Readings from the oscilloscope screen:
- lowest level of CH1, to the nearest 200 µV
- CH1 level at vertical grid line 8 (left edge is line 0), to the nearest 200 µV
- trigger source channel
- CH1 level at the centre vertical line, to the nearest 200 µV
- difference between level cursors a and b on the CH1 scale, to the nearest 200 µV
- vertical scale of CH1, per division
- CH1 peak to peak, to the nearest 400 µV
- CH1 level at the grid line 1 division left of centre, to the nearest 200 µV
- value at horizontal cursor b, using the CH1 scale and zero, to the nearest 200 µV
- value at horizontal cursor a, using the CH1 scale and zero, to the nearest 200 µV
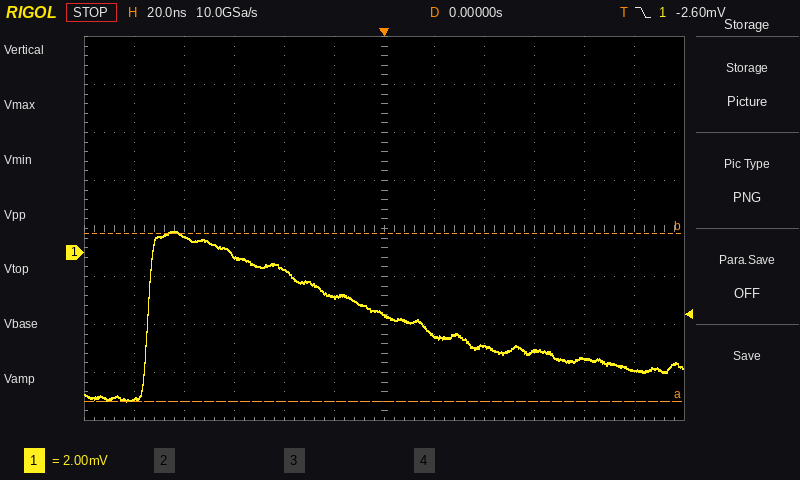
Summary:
-6.2 mV
-4.0 mV
CH1
-2.6 mV
7.0 mV
2 mV
7.2 mV
-1.8 mV
800 µV
-6.2 mV
